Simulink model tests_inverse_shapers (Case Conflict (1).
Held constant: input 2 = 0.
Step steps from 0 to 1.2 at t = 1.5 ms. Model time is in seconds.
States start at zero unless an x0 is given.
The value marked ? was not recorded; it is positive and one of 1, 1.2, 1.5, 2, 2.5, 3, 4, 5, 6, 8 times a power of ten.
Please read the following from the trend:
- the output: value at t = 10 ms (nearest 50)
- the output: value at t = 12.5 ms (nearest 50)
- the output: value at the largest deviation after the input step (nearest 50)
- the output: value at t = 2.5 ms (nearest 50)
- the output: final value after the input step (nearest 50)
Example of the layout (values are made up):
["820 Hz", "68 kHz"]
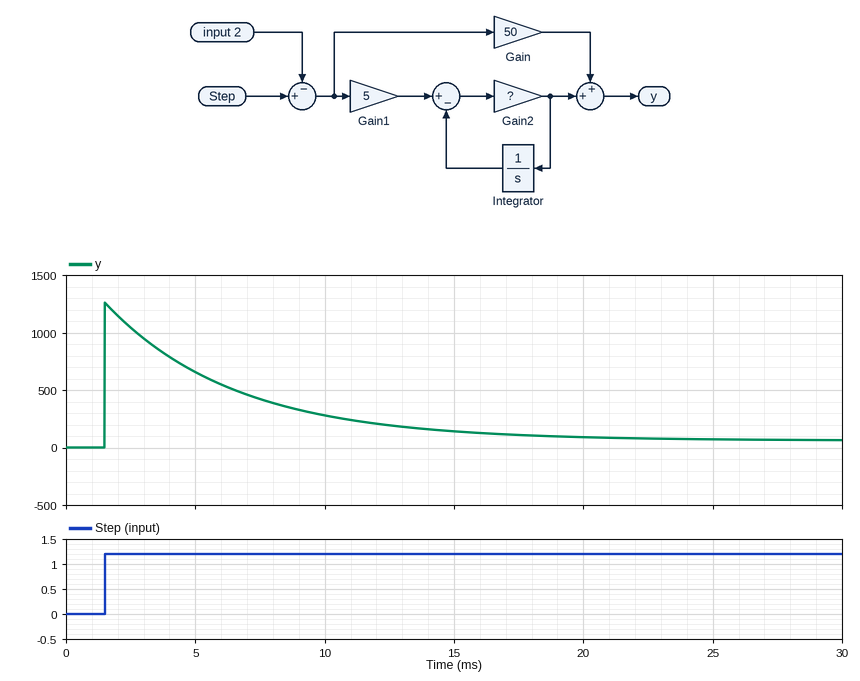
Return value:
["300", "200", "1250", "1050", "50"]
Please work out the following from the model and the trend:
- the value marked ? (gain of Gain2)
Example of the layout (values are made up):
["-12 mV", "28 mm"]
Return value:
["200"]
